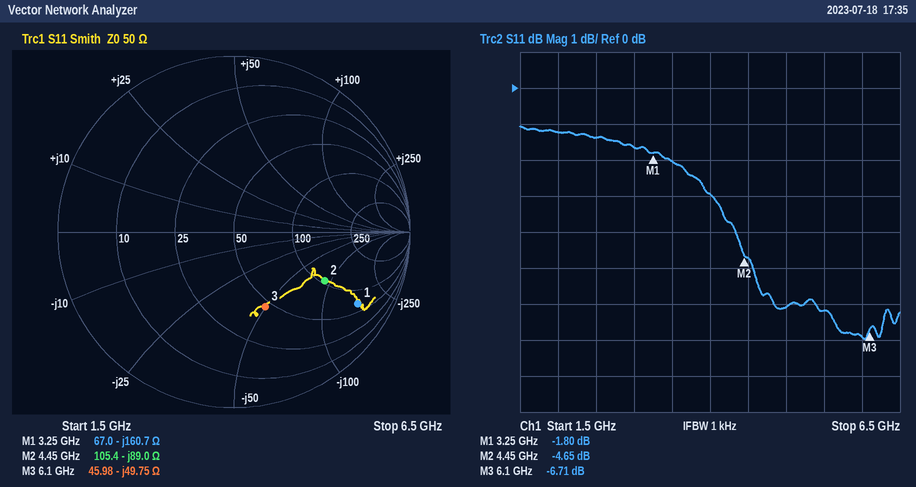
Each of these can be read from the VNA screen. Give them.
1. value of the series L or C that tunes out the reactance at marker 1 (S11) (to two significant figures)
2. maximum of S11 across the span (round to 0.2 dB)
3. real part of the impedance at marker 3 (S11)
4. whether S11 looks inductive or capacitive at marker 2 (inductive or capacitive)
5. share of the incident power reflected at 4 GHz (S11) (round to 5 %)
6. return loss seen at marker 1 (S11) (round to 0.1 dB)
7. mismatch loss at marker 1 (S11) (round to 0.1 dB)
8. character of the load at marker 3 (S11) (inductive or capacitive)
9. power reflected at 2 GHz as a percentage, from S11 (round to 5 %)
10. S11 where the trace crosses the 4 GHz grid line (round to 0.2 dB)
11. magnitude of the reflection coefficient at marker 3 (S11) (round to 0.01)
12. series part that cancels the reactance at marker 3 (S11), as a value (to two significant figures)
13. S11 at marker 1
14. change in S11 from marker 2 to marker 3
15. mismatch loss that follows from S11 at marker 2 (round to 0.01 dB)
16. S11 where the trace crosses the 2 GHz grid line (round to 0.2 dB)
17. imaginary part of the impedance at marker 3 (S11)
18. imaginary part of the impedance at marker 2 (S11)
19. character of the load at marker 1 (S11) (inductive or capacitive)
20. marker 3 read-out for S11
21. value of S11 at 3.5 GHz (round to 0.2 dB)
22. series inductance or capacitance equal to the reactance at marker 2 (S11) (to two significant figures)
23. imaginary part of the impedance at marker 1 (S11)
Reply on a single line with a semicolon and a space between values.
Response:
7.9 nH; -1.0 dB; 45.98 Ω; capacitive; 50 %; 1.8 dB; 4.7 dB; capacitive; 75 %; -3.0 dB; 0.46; 1.3 nH; -1.80 dB; -2.06 dB; 1.82 dB; -1.2 dB; -49.75 Ω; -89.0 Ω; capacitive; -6.71 dB; -2.0 dB; 400 fF; -160.7 Ω
